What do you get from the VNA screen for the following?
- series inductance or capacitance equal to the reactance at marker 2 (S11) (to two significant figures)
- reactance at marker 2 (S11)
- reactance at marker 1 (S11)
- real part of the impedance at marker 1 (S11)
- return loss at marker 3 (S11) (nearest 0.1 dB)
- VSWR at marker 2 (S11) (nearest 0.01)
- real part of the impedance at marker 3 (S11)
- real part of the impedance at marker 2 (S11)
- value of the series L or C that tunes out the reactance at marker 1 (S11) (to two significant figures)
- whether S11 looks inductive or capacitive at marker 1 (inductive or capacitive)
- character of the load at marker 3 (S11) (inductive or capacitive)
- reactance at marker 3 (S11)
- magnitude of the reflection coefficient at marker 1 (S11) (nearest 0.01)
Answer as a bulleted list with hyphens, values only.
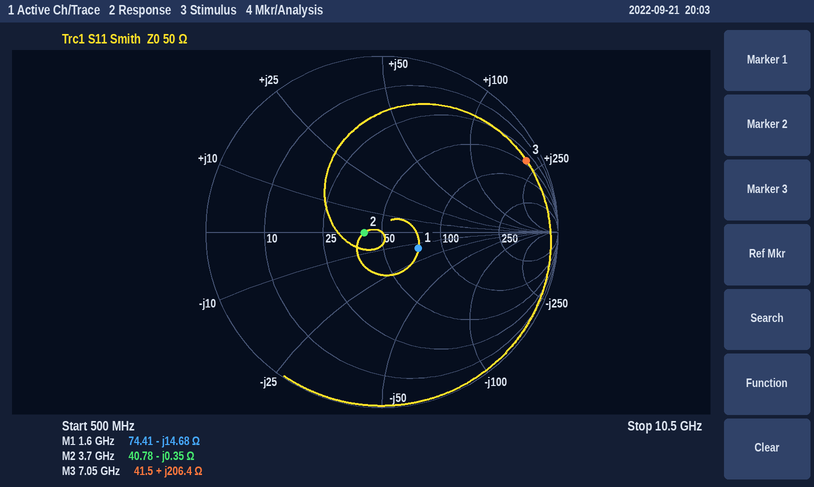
- 120 pF
- -0.35 Ω
- -14.68 Ω
- 74.41 Ω
- 0.8 dB
- 1.23
- 41.5 Ω
- 40.78 Ω
- 1.5 nH
- capacitive
- inductive
- +206.4 Ω
- 0.23
